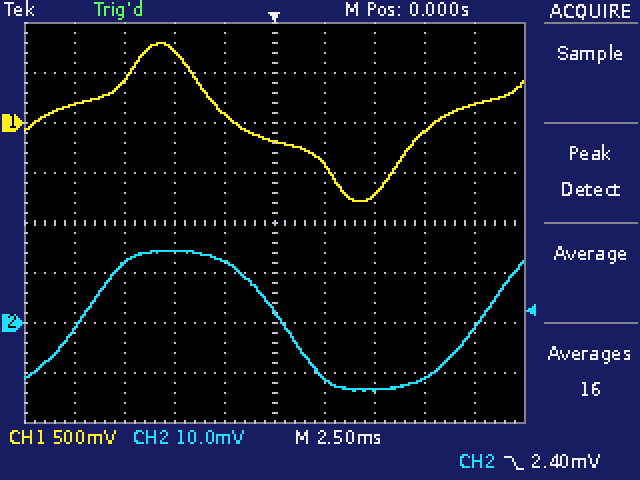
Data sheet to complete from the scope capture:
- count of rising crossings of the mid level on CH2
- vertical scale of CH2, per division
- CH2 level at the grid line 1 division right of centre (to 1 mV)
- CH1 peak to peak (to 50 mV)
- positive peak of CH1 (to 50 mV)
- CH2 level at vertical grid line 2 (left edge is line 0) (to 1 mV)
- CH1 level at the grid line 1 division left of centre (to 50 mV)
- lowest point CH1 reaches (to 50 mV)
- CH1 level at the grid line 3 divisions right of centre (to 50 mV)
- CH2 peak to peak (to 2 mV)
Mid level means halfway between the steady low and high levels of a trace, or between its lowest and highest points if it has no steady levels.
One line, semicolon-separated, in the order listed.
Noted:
2; 10 mV; -11 mV; 1.60 V; 800 mV; 12 mV; 100 mV; -800 mV; -100 mV; 28 mV
